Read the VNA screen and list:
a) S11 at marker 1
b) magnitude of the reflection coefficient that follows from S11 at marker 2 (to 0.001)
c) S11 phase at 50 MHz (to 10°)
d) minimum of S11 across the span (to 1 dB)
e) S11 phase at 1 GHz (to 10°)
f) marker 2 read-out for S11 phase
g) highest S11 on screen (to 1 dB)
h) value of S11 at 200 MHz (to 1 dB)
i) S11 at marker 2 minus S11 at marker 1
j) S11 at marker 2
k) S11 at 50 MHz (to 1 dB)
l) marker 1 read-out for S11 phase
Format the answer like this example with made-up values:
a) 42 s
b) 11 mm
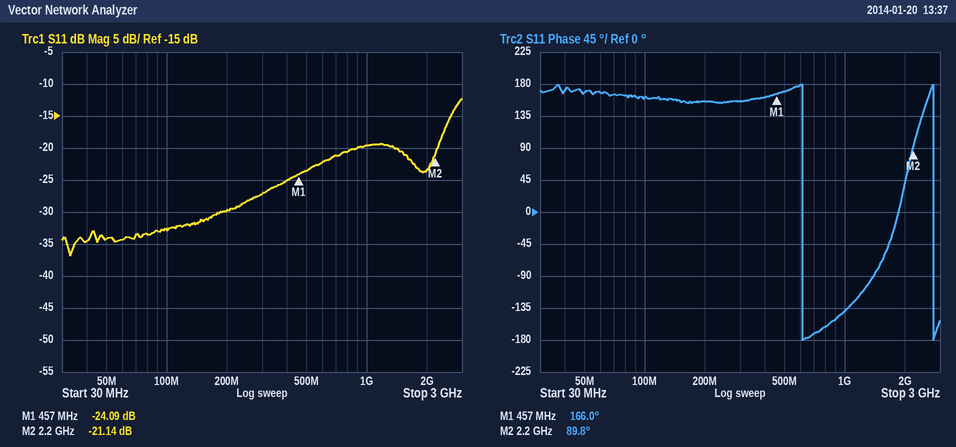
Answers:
a) -24.09 dB
b) 0.088
c) 170°
d) -37 dB
e) -140°
f) 89.8°
g) -12 dB
h) -30 dB
i) 2.95 dB
j) -21.14 dB
k) -34 dB
l) 166.0°
